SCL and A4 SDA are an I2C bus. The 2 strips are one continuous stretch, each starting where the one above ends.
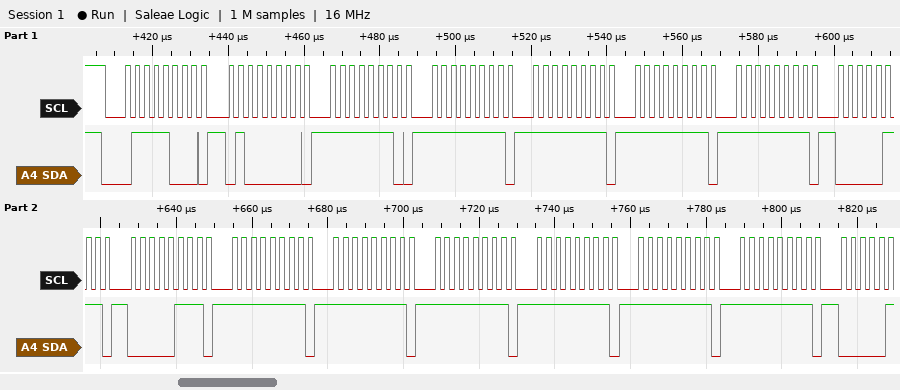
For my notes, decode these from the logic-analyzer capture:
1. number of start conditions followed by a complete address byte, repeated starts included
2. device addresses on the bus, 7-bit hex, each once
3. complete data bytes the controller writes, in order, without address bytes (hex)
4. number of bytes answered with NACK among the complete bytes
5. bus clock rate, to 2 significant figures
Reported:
1
0x3C
40 FE FF FF FF FF 07 07 FF FF FF FF FF FF
0
400 kHz
